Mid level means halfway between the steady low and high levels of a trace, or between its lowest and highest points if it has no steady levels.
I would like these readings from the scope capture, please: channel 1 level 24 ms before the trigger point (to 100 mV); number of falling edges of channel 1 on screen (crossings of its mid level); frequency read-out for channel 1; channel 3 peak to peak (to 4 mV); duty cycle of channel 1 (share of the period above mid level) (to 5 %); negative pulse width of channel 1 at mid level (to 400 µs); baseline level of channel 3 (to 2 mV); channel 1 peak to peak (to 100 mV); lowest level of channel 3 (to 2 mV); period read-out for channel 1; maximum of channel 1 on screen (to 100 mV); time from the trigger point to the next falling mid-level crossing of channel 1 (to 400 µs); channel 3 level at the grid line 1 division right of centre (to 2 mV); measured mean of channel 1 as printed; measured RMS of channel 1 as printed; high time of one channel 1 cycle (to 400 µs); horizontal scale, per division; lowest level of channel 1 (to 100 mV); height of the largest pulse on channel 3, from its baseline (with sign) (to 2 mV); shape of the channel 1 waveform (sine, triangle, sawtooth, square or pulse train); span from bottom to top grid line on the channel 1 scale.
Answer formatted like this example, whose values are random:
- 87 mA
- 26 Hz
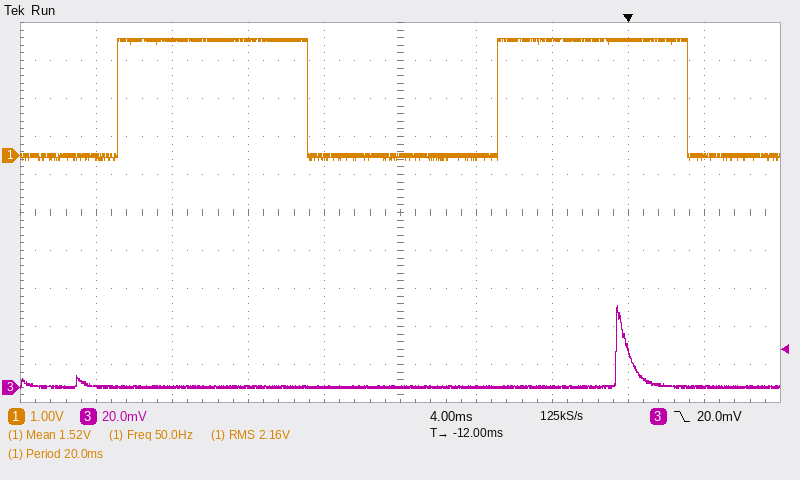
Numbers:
- 3.0 V
- 2
- 50.0 Hz
- 44 mV
- 50 %
- 10.0 ms
- 0 mV
- 3.2 V
- 0 mV
- 20.0 ms
- 3.1 V
- 3.2 ms
- 0 mV
- 1.52 V
- 2.16 V
- 10.0 ms
- 4 ms
- -100 mV
- +42 mV
- square
- 10 V
